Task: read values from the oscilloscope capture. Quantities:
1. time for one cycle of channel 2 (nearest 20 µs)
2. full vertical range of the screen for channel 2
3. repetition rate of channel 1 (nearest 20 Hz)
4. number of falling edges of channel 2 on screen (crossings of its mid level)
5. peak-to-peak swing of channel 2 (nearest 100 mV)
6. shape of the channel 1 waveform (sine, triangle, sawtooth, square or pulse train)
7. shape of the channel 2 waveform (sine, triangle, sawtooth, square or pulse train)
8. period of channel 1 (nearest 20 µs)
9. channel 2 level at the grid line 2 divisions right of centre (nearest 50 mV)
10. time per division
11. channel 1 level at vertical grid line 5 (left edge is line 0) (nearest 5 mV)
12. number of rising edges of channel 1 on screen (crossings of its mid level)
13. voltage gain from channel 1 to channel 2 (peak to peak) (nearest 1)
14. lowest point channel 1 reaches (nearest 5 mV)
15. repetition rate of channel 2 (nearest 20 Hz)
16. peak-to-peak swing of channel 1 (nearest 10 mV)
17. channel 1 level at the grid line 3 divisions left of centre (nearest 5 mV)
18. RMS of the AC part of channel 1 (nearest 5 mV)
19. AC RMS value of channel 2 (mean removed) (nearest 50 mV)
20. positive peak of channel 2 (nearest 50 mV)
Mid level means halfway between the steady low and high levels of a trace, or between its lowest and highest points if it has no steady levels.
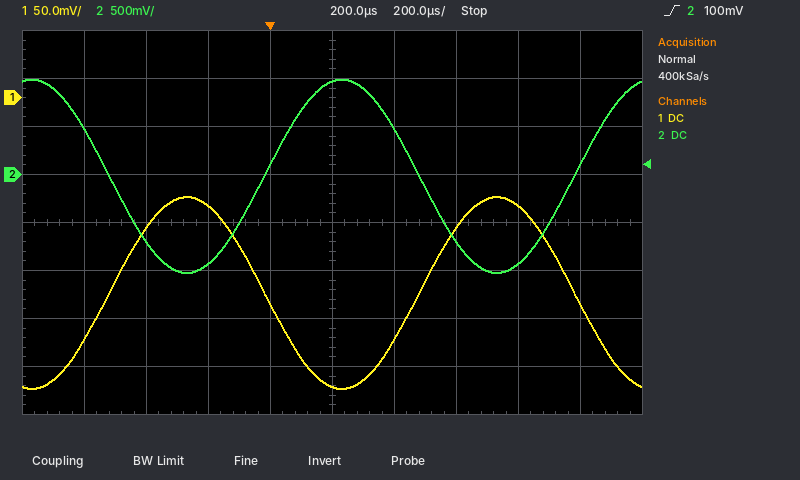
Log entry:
1.00 ms
4 V
1.00 kHz
2
2.00 V
sine
sine
1.00 ms
-700 mV
200 µs
-300 mV
2
10
-305 mV
1.00 kHz
200 mV
-135 mV
70 mV
700 mV
1.00 V
